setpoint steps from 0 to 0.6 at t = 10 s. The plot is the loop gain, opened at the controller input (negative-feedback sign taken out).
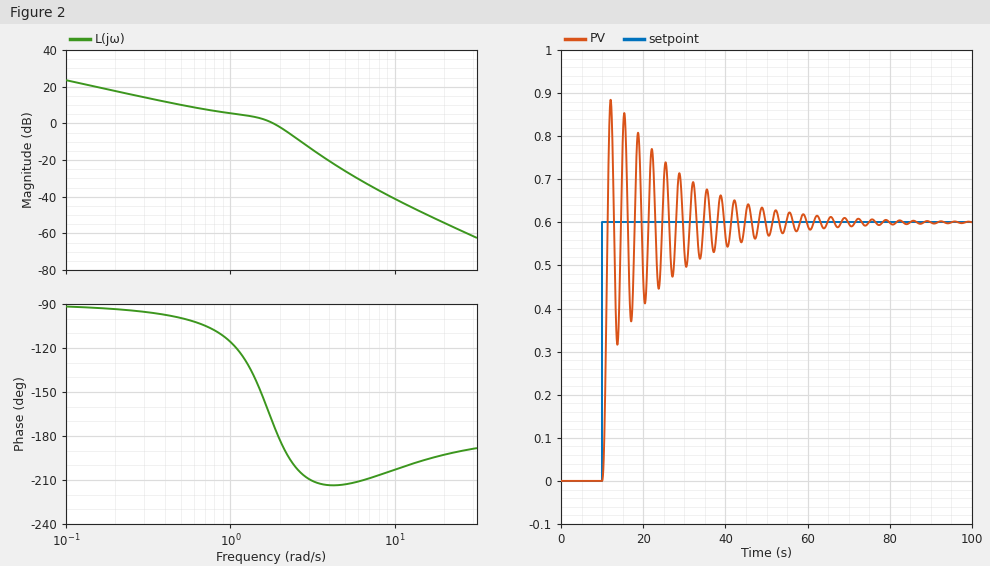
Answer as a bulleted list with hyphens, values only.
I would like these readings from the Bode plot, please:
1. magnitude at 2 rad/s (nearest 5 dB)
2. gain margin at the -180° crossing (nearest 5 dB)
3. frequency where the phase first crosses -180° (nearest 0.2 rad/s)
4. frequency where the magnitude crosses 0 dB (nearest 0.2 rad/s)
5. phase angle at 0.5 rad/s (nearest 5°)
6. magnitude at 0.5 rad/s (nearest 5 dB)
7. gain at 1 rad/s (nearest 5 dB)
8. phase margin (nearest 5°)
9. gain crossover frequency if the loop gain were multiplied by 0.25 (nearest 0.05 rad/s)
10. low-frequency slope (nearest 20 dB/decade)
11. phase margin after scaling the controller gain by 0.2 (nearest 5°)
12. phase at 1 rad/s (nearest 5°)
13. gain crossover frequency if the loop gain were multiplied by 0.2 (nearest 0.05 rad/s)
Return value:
- 0 dB
- 0 dB
- 2.0 rad/s
- 1.8 rad/s
- -100°
- 10 dB
- 5 dB
- 10°
- 0.40 rad/s
- -20 dB/decade
- 85°
- -115°
- 0.30 rad/s
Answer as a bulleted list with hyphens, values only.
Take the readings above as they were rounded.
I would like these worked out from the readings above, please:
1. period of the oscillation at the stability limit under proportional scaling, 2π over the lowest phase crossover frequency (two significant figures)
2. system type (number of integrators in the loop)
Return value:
- 3.1 s
- 1
